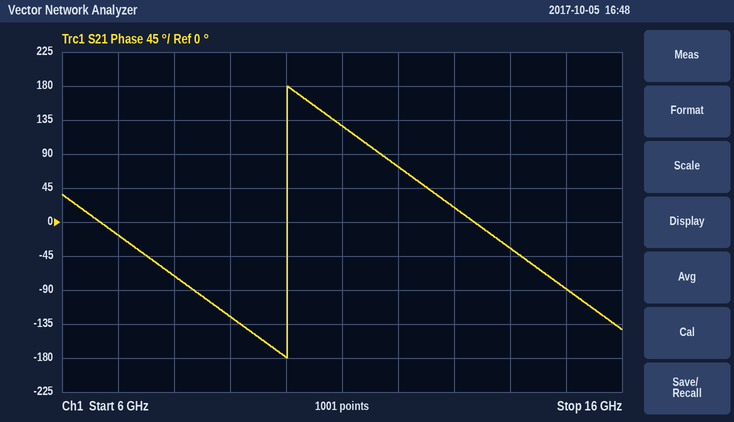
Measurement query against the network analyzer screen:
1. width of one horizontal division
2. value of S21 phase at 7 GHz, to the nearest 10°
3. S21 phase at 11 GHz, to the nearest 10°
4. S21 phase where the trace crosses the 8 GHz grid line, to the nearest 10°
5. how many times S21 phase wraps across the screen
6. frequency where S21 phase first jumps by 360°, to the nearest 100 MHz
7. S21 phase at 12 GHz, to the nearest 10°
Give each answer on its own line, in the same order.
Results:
1 GHz
-20°
130°
-70°
1
10.0 GHz
70°
